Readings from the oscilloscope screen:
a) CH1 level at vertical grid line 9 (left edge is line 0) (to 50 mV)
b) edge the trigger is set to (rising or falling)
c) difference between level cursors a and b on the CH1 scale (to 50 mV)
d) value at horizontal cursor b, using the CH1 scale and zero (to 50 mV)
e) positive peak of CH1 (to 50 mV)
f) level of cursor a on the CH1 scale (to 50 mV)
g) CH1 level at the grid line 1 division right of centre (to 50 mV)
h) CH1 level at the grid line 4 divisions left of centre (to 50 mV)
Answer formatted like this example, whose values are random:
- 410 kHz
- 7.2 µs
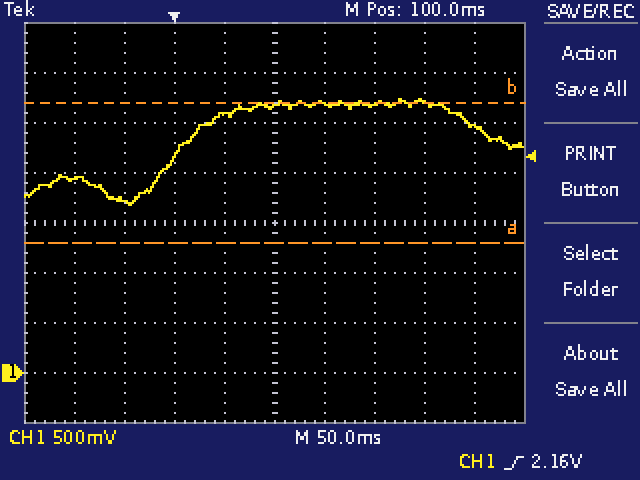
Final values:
- 2.45 V
- rising
- 1.40 V
- 2.70 V
- 2.75 V
- 1.30 V
- 2.70 V
- 1.95 V
